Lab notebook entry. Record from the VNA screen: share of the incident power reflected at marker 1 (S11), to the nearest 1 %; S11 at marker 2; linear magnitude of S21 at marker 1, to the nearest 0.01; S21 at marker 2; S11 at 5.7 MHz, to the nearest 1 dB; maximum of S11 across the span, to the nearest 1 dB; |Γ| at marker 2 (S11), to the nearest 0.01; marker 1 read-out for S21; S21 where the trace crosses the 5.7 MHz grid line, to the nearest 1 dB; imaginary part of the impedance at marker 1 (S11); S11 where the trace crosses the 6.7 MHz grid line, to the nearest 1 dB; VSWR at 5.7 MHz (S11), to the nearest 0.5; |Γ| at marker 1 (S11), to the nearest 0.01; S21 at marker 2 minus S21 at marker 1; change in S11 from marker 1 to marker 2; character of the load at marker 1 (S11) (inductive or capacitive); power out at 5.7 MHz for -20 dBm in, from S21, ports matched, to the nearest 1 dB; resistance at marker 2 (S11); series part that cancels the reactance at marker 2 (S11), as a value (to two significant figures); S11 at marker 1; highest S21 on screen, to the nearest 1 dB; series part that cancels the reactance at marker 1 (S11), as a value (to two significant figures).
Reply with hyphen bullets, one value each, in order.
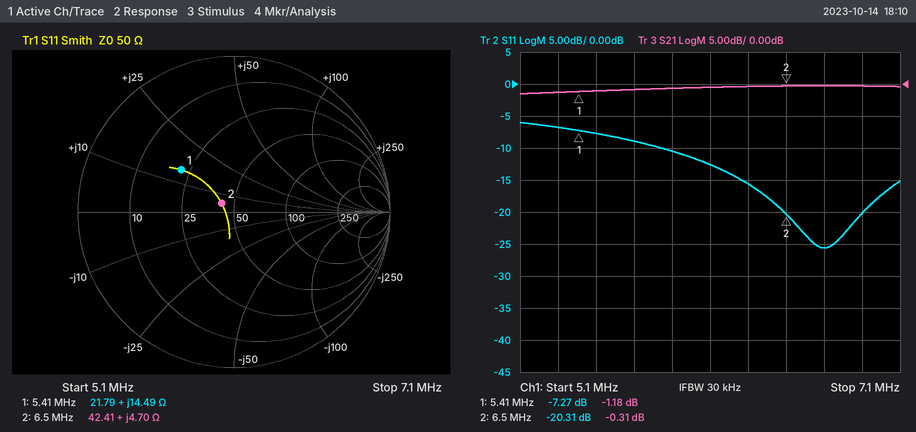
- 19 %
- -20.31 dB
- 0.87
- -0.31 dB
- -9 dB
- -6 dB
- 0.10
- -1.18 dB
- -1 dB
- +14.49 Ω
- -26 dB
- 2.0
- 0.43
- 0.87 dB
- -13.04 dB
- inductive
- -21 dBm
- 42.41 Ω
- 5.2 nF
- -7.27 dB
- 0 dB
- 2.0 nF
